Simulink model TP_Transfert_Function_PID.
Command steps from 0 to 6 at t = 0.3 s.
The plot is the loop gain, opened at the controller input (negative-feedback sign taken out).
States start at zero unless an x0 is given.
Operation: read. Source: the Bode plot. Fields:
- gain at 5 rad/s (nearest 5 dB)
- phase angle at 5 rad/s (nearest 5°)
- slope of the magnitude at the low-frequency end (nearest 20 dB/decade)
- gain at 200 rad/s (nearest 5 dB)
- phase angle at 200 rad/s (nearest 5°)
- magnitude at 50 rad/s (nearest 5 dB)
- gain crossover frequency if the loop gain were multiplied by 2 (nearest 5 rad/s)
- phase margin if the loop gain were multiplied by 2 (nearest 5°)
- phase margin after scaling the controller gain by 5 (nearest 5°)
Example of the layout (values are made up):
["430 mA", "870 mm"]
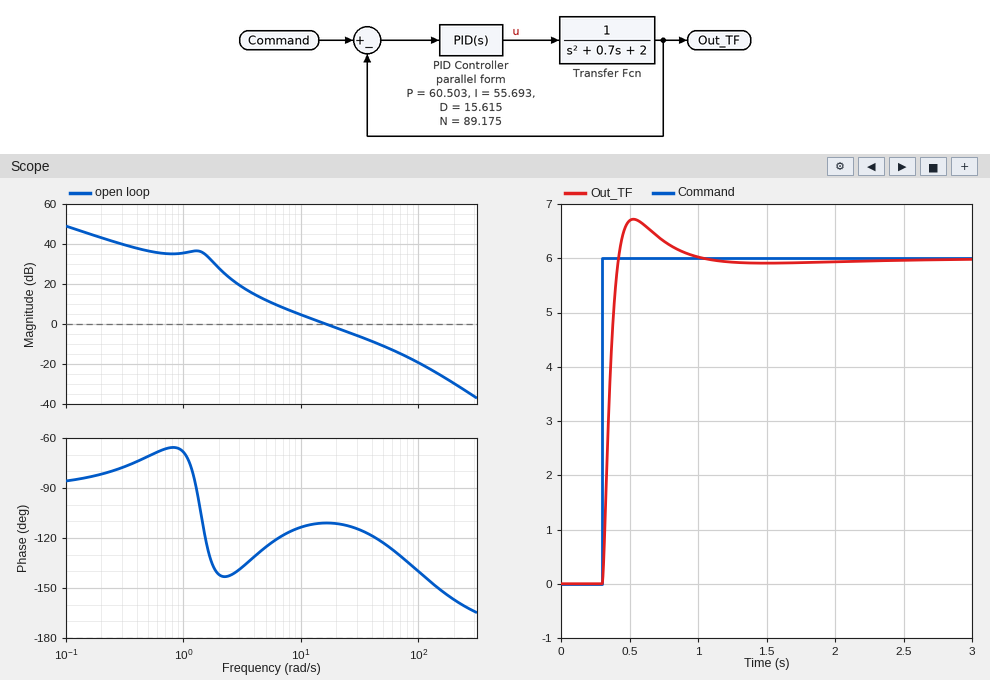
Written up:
["10 dB", "-125°", "-20 dB/decade", "-30 dB", "-155°", "-10 dB", "30 rad/s", "65°", "50°"]
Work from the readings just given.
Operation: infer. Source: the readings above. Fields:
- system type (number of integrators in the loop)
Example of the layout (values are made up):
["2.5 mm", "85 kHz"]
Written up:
["1"]
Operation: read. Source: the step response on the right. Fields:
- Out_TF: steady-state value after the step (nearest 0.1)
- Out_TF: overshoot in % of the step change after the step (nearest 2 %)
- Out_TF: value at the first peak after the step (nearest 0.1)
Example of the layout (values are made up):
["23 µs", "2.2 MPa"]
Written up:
["6.0", "12 %", "6.7"]
